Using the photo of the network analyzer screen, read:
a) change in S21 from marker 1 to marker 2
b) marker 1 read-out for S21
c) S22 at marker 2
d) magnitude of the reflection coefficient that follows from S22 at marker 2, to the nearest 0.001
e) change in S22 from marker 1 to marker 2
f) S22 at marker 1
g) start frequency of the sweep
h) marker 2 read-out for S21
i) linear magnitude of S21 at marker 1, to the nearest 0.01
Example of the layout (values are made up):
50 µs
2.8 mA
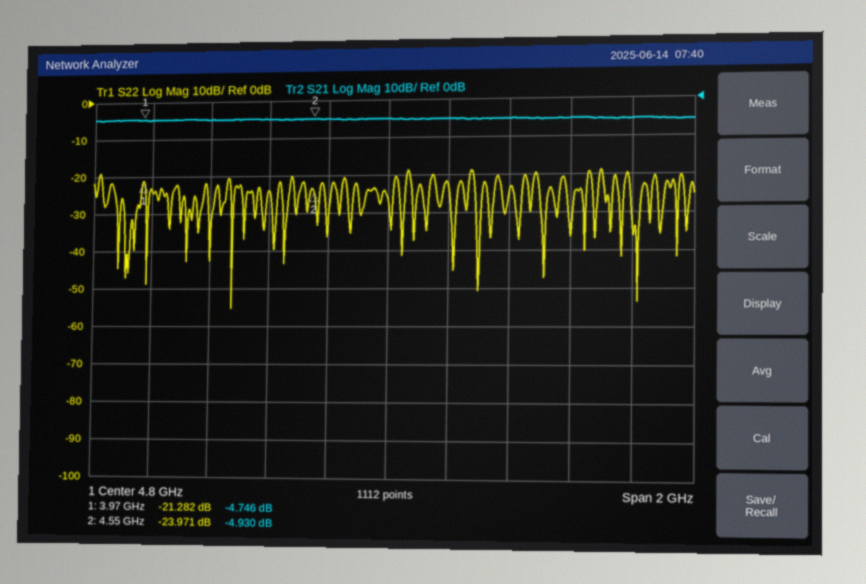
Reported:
-0.184 dB
-4.746 dB
-23.971 dB
0.063
-2.689 dB
-21.282 dB
3.8 GHz
-4.930 dB
0.58
